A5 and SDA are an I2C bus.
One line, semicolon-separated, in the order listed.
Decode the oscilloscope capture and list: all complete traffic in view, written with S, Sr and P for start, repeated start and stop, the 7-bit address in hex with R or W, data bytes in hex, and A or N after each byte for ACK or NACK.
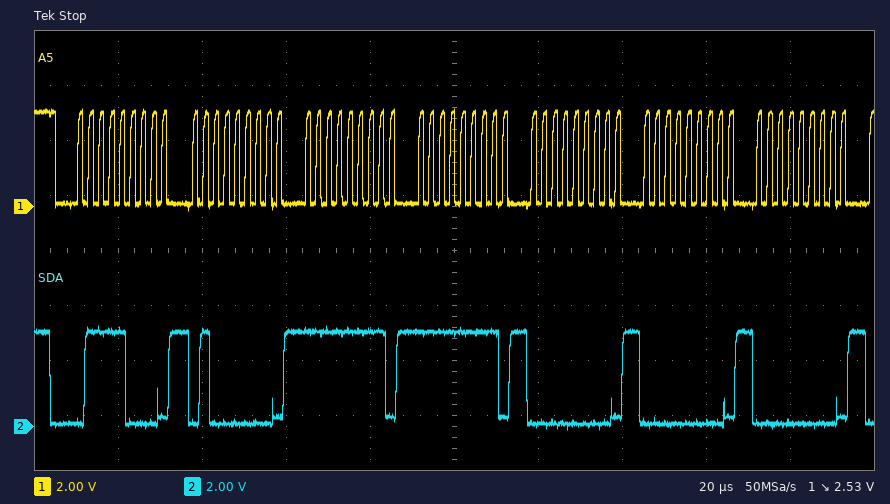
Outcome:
S 3CW A 40 A FF A FF A 00 A 00 A 00 A
